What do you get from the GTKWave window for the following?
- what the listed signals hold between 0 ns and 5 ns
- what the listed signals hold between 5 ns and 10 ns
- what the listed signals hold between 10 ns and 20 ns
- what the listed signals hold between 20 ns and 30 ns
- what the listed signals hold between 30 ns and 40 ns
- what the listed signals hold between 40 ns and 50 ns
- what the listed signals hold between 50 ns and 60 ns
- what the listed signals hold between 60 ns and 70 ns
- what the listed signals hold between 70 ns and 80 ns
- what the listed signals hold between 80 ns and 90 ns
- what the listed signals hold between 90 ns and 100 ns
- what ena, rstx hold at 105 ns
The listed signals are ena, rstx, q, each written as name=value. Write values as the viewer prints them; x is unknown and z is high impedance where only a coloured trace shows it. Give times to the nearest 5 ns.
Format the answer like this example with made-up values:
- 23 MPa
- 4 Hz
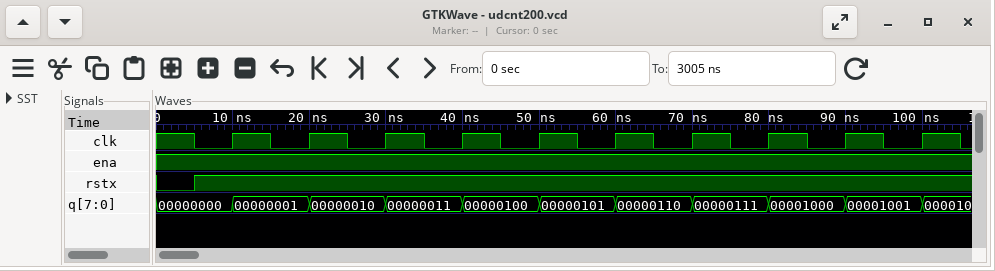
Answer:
- ena=1, rstx=0, q=00000000
- ena=1, rstx=1, q=00000000
- ena=1, rstx=1, q=00000001
- ena=1, rstx=1, q=00000010
- ena=1, rstx=1, q=00000011
- ena=1, rstx=1, q=00000100
- ena=1, rstx=1, q=00000101
- ena=1, rstx=1, q=00000110
- ena=1, rstx=1, q=00000111
- ena=1, rstx=1, q=00001000
- ena=1, rstx=1, q=00001001
- ena=1, rstx=1
